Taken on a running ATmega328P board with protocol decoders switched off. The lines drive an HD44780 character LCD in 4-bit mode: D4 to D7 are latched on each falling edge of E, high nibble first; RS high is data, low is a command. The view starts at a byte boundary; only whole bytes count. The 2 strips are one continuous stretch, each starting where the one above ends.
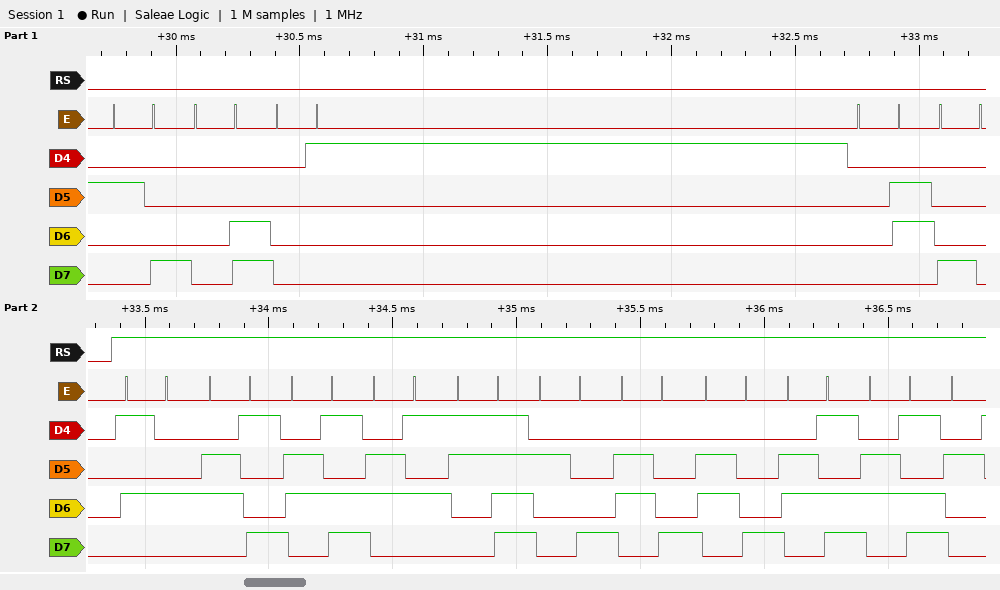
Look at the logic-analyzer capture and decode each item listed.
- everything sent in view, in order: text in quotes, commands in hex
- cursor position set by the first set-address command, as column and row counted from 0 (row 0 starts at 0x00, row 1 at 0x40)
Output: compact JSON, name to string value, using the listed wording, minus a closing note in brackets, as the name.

{"everything sent in view, in order: text in quotes, commands in hex": "0x28 0x0C 0x01 0x06 0x80 \"Time?(hhmm\"", "cursor position set by the first set-address command, as column and row counted from 0": "column 0, row 0"}
